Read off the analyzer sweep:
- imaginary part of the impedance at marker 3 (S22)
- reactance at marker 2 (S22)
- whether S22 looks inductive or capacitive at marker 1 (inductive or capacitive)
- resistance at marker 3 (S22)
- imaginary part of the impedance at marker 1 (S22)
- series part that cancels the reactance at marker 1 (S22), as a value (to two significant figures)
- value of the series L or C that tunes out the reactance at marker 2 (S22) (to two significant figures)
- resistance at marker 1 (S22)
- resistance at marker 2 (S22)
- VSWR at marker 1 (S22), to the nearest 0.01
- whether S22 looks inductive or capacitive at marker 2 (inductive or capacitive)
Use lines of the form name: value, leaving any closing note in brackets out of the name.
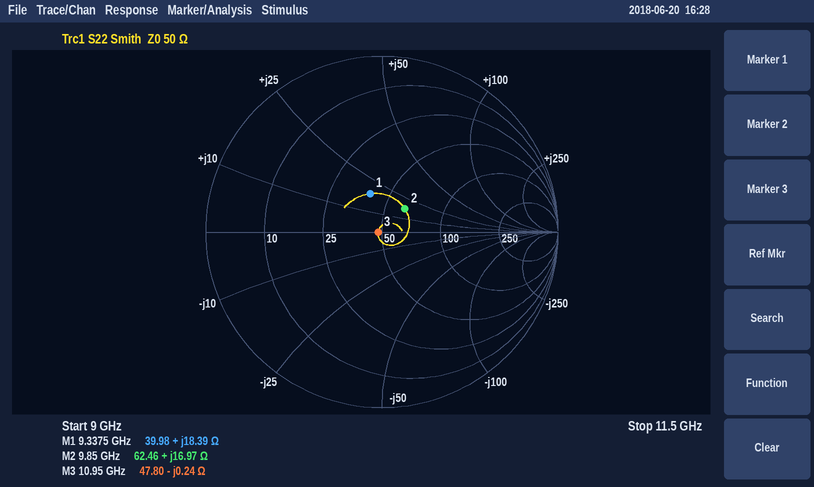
imaginary part of the impedance at marker 3: -0.24 Ω
reactance at marker 2: +16.97 Ω
whether S22 looks inductive or capacitive at marker 1: inductive
resistance at marker 3: 47.80 Ω
imaginary part of the impedance at marker 1: +18.39 Ω
series part that cancels the reactance at marker 1 (S22), as a value: 930 fF
value of the series L or C that tunes out the reactance at marker 2 (S22): 950 fF
resistance at marker 1: 39.98 Ω
resistance at marker 2: 62.46 Ω
VSWR at marker 1 (S22), to the nearest 0.01: 1.59
whether S22 looks inductive or capacitive at marker 2: inductive
